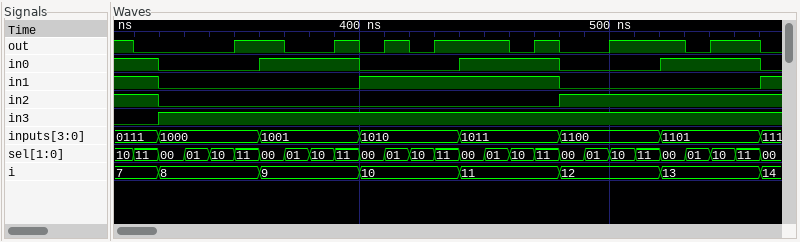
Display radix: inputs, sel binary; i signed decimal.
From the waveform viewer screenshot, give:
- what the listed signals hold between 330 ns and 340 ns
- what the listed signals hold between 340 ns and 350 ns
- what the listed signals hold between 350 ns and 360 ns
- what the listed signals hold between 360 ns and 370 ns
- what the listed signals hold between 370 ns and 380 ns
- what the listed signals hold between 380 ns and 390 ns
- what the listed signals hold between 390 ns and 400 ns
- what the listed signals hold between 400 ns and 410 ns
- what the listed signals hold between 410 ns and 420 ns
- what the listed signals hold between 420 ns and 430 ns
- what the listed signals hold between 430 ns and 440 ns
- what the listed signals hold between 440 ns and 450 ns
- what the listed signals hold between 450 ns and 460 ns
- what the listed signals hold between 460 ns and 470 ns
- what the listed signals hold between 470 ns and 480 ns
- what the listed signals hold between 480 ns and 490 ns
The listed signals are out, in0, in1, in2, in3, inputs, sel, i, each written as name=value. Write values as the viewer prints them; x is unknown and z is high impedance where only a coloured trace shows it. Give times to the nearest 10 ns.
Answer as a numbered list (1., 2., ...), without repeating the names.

1. out=0, in0=0, in1=0, in2=0, in3=1, inputs=1000, sel=01, i=8
2. out=0, in0=0, in1=0, in2=0, in3=1, inputs=1000, sel=10, i=8
3. out=1, in0=0, in1=0, in2=0, in3=1, inputs=1000, sel=11, i=8
4. out=1, in0=1, in1=0, in2=0, in3=1, inputs=1001, sel=00, i=9
5. out=0, in0=1, in1=0, in2=0, in3=1, inputs=1001, sel=01, i=9
6. out=0, in0=1, in1=0, in2=0, in3=1, inputs=1001, sel=10, i=9
7. out=1, in0=1, in1=0, in2=0, in3=1, inputs=1001, sel=11, i=9
8. out=0, in0=0, in1=1, in2=0, in3=1, inputs=1010, sel=00, i=10
9. out=1, in0=0, in1=1, in2=0, in3=1, inputs=1010, sel=01, i=10
10. out=0, in0=0, in1=1, in2=0, in3=1, inputs=1010, sel=10, i=10
11. out=1, in0=0, in1=1, in2=0, in3=1, inputs=1010, sel=11, i=10
12. out=1, in0=1, in1=1, in2=0, in3=1, inputs=1011, sel=00, i=11
13. out=1, in0=1, in1=1, in2=0, in3=1, inputs=1011, sel=01, i=11
14. out=0, in0=1, in1=1, in2=0, in3=1, inputs=1011, sel=10, i=11
15. out=1, in0=1, in1=1, in2=0, in3=1, inputs=1011, sel=11, i=11
16. out=0, in0=0, in1=0, in2=1, in3=1, inputs=1100, sel=00, i=12
